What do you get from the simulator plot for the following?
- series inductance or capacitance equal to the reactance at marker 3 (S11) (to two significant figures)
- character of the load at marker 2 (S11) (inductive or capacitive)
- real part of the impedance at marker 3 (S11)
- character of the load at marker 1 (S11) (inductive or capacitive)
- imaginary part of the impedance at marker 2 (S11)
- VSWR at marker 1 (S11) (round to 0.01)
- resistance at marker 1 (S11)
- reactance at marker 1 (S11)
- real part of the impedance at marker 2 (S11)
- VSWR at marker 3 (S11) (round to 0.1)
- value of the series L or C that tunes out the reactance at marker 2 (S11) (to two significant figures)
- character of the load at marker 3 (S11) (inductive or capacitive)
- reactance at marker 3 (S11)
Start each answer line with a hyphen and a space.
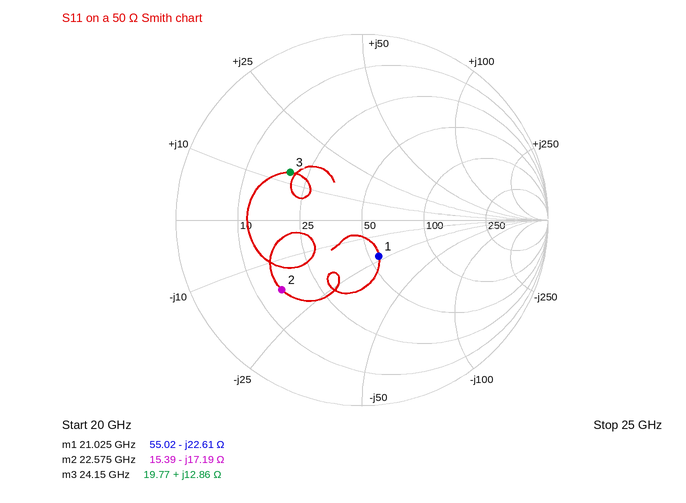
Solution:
- 85 pH
- capacitive
- 19.77 Ω
- capacitive
- -17.19 Ω
- 1.55
- 55.02 Ω
- -22.61 Ω
- 15.39 Ω
- 2.7
- 120 pH
- inductive
- +12.86 Ω
